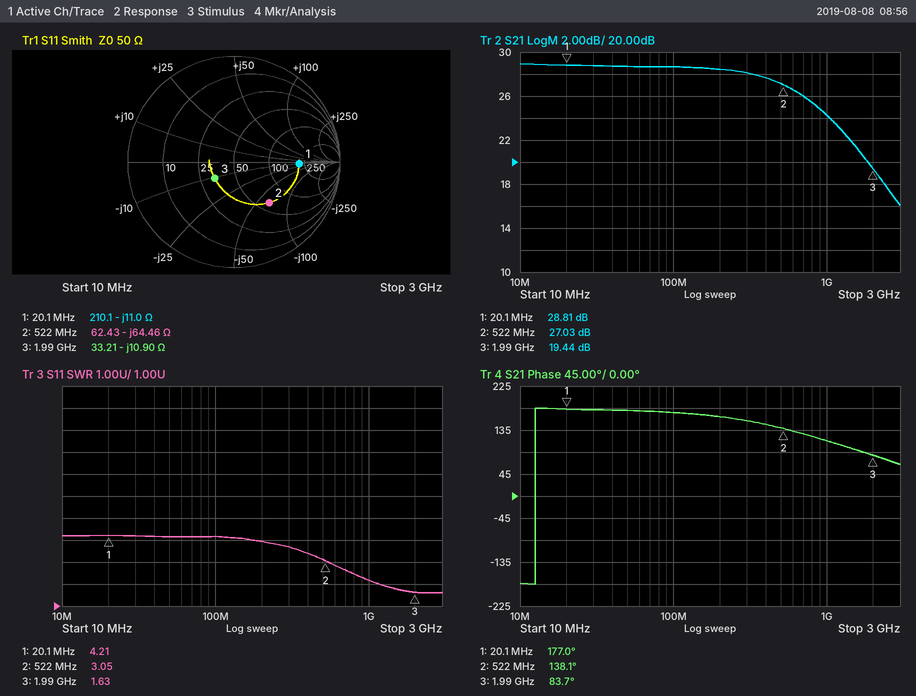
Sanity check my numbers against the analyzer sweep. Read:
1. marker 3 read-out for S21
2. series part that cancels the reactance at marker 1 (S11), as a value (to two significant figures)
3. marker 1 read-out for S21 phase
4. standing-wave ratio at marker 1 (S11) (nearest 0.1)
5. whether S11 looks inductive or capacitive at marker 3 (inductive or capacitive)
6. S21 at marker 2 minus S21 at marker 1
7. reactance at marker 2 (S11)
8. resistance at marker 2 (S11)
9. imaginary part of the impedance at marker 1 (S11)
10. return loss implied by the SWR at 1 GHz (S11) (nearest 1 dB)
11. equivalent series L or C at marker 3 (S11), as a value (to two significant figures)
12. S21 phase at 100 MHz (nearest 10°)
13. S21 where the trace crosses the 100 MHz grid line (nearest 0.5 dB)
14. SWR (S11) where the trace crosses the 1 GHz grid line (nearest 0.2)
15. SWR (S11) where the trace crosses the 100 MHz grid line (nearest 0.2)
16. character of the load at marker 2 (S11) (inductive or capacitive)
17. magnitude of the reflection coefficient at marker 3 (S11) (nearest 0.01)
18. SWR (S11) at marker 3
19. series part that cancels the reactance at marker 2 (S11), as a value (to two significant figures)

19.44 dB
87 nH
177.0°
4.2
capacitive
-1.78 dB
-64.46 Ω
62.43 Ω
-11.0 Ω
9 dB
7.3 pF
170°
28.5 dB
2.2
4.2
capacitive
0.24
1.63
20 nH
